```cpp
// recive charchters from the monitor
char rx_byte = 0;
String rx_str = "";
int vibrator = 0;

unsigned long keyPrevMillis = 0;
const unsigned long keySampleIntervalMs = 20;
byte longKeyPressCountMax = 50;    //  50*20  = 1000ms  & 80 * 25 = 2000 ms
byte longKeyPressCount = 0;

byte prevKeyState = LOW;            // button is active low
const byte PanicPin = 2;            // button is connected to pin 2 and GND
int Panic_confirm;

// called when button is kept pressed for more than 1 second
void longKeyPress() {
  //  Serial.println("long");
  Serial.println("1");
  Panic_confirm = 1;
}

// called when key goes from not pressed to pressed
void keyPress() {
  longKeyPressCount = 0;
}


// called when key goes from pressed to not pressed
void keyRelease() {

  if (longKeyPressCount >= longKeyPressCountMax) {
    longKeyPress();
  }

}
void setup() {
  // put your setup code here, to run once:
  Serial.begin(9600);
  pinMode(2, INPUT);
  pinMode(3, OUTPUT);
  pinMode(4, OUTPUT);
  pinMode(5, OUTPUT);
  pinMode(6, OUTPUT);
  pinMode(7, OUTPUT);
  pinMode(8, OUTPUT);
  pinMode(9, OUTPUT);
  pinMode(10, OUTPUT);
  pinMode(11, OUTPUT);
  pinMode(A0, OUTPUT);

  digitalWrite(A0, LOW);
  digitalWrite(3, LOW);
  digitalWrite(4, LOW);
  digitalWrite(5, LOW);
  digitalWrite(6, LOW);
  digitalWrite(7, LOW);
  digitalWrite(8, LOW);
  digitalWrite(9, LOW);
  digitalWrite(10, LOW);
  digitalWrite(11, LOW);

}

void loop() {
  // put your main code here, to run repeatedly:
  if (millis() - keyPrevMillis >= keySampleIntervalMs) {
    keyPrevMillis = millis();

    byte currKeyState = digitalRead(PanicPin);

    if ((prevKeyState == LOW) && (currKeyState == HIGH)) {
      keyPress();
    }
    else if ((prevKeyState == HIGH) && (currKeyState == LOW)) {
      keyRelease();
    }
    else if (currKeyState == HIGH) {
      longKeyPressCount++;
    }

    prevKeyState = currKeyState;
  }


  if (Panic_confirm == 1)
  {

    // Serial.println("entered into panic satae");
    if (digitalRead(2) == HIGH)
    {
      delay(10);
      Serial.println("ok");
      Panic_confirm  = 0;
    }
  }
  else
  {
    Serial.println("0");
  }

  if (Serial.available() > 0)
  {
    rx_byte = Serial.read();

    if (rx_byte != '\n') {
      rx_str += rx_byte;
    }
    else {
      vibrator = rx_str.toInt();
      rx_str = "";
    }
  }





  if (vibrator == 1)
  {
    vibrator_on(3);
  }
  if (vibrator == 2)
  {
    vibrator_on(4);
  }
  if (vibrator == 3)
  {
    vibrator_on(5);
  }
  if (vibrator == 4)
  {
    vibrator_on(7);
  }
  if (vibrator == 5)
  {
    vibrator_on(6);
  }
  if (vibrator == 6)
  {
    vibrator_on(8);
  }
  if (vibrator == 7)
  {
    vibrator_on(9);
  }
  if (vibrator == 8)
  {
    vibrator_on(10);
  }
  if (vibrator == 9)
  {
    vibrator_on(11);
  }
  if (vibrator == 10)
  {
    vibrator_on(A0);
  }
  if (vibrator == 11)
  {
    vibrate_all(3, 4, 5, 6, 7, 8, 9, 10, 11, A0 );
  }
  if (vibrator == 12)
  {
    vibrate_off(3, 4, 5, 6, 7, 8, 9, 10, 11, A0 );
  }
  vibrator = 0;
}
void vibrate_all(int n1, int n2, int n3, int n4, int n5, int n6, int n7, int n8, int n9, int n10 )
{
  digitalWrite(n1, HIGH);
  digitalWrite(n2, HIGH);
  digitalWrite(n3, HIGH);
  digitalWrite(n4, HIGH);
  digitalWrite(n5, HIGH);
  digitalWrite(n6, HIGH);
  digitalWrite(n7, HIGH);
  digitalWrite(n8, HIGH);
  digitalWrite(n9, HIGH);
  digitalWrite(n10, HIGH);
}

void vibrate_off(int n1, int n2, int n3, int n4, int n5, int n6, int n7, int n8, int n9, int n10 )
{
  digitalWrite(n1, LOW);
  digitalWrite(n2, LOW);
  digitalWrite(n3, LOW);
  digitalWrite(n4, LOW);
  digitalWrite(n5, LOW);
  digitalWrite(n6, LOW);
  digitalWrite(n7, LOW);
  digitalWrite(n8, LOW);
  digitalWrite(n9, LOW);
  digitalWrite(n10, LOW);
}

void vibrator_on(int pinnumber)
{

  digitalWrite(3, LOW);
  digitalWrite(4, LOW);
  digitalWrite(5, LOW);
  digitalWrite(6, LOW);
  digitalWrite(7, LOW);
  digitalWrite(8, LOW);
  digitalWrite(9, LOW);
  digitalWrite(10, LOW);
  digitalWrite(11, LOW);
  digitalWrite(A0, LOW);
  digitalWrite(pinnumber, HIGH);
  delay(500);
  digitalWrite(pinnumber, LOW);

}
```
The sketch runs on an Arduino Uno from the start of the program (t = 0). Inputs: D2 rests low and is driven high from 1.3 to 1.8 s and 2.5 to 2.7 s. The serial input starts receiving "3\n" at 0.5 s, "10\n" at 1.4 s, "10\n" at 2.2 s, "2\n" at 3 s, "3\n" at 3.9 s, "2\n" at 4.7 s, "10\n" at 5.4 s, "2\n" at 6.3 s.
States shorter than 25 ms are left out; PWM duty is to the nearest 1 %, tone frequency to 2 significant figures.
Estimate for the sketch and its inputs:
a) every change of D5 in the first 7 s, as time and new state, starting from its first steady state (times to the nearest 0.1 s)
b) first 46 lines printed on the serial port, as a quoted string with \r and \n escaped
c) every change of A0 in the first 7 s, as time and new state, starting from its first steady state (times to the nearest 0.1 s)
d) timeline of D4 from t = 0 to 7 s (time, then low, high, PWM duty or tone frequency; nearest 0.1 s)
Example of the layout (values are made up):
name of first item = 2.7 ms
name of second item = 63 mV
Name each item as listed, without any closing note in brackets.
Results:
every change of D5 in the first 7 s, as time and new state, starting from its first steady state = 0 s low; 0.5 s high; 1 s low; 3.9 s high; 4.4 s low
first 46 lines printed on the serial port, as a quoted string with \r and \n escaped = "0\r\n0\r\n0\r\n0\r\n0\r\n0\r\n0\r\n0\r\n0\r\n0\r\n0\r\n0\r\n0\r\n0\r\n0\r\n0\r\n0\r\n0\r\n0\r\n0\r\n0\r\n0\r\n0\r\n0\r\n0\r\n0\r\n0\r\n0\r\n0\r\n0\r\n0\r\n0\r\n0\r\n0\r\n0\r\n0\r\n0\r\n0\r\n0\r\n0\r\n0\r\n0\r\n0\r\n0\r\n0\r\n0\r\n"
every change of A0 in the first 7 s, as time and new state, starting from its first steady state = 0 s low; 1.4 s high; 1.9 s low; 2.2 s high; 2.7 s low; 5.4 s high; 5.9 s low
timeline of D4 from t = 0 to 7 s = 0 s low; 3 s high; 3.5 s low; 4.7 s high; 5.2 s low; 6.3 s high; 6.8 s low
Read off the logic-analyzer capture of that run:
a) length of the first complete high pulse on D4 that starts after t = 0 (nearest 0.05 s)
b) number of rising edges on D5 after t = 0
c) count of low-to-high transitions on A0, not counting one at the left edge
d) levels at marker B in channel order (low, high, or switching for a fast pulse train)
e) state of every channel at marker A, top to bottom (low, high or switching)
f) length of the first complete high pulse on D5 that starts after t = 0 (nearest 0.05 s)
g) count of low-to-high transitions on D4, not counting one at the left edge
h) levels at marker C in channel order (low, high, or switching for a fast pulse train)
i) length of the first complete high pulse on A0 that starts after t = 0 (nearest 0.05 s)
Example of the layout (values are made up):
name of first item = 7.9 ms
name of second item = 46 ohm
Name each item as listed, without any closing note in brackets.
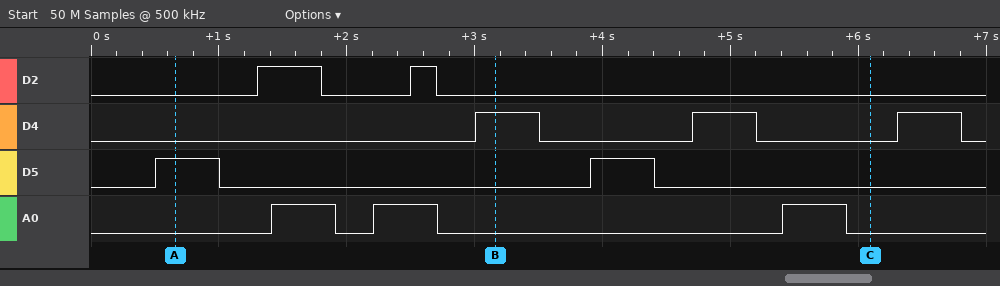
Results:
length of the first complete high pulse on D4 that starts after t = 0 = 0.50 s
number of rising edges on D5 after t = 0 = 2
count of low-to-high transitions on A0, not counting one at the left edge = 3
levels at marker B in channel order = D2 low, D4 high, D5 low, A0 low
state of every channel at marker A, top to bottom = D2 low, D4 low, D5 high, A0 low
length of the first complete high pulse on D5 that starts after t = 0 = 0.50 s
count of low-to-high transitions on D4, not counting one at the left edge = 3
levels at marker C in channel order = D2 low, D4 low, D5 low, A0 low
length of the first complete high pulse on A0 that starts after t = 0 = 0.50 s
